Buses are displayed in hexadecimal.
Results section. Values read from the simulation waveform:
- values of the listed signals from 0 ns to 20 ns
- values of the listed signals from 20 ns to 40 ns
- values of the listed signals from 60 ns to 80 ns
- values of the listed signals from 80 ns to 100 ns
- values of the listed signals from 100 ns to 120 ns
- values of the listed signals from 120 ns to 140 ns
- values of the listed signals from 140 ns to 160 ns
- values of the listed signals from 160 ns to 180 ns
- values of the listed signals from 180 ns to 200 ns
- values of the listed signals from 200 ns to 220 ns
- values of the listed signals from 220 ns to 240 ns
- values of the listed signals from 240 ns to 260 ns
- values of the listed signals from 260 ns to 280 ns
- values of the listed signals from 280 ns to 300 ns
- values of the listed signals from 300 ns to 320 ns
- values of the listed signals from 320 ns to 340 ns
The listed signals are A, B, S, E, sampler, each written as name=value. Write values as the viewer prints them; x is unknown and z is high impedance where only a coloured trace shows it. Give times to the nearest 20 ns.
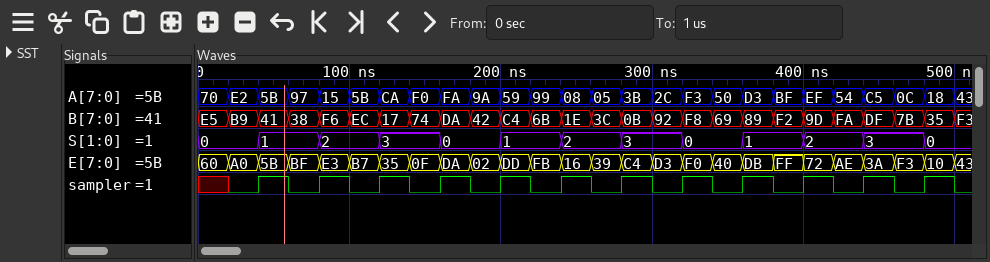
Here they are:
A=70, B=E5, S=0, E=60, sampler=x
A=E2, B=B9, S=0, E=A0, sampler=0
A=97, B=38, S=1, E=BF, sampler=0
A=15, B=F6, S=2, E=E3, sampler=1
A=5B, B=EC, S=2, E=B7, sampler=0
A=CA, B=17, S=3, E=35, sampler=1
A=F0, B=74, S=3, E=0F, sampler=0
A=FA, B=DA, S=0, E=DA, sampler=1
A=9A, B=42, S=0, E=02, sampler=0
A=59, B=C4, S=1, E=DD, sampler=1
A=99, B=6B, S=1, E=FB, sampler=0
A=08, B=1E, S=2, E=16, sampler=1
A=05, B=3C, S=2, E=39, sampler=0
A=3B, B=0B, S=3, E=C4, sampler=1
A=2C, B=92, S=3, E=D3, sampler=0
A=F3, B=F8, S=0, E=F0, sampler=1
